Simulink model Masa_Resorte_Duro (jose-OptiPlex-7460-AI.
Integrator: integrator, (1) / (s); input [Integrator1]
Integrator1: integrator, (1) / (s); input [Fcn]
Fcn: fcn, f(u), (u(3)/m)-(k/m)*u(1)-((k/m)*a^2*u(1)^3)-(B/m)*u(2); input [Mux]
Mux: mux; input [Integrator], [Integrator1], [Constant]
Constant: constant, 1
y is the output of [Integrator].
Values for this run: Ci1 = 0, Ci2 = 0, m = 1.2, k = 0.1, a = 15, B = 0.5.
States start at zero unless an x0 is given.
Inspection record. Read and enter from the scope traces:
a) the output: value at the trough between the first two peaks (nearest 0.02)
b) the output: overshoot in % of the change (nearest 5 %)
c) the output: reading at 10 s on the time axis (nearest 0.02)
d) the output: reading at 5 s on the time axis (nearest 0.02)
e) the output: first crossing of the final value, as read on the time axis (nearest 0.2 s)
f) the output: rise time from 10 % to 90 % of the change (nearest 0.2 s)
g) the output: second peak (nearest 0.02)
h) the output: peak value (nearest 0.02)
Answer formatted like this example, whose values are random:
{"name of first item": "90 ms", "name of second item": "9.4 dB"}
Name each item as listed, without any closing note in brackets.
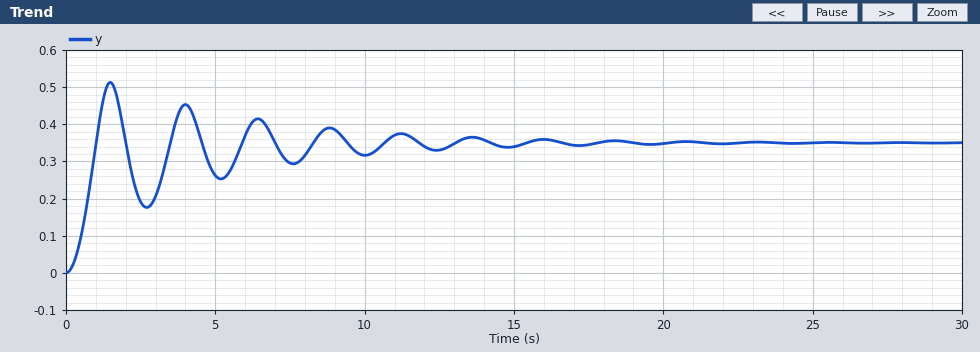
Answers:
{"the output: value at the trough between the first two peaks": "0.18", "the output: overshoot in % of the change": "45 %", "the output: reading at 10 s on the time axis": "0.32", "the output: reading at 5 s on the time axis": "0.26", "the output: first crossing of the final value, as read on the time axis": "1.0 s", "the output: rise time from 10 % to 90 % of the change": "0.6 s", "the output: second peak": "0.46", "the output: peak value": "0.52"}
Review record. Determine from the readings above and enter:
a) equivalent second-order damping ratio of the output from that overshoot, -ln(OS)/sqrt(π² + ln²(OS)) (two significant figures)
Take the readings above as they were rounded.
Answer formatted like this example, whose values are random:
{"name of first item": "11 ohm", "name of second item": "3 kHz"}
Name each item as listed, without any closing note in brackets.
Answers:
{"equivalent second-order damping ratio of the output from that overshoot, -ln(OS)/sqrt(π² + ln²(OS))": "0.25"}
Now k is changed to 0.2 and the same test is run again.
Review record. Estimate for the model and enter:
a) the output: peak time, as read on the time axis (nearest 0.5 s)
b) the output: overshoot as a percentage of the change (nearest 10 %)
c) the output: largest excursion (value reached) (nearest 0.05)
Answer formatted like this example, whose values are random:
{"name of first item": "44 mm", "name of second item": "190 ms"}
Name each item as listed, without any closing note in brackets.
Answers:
{"the output: peak time, as read on the time axis": "1.5 s", "the output: overshoot as a percentage of the change": "50 %", "the output: largest excursion (value reached)": "0.40"}
